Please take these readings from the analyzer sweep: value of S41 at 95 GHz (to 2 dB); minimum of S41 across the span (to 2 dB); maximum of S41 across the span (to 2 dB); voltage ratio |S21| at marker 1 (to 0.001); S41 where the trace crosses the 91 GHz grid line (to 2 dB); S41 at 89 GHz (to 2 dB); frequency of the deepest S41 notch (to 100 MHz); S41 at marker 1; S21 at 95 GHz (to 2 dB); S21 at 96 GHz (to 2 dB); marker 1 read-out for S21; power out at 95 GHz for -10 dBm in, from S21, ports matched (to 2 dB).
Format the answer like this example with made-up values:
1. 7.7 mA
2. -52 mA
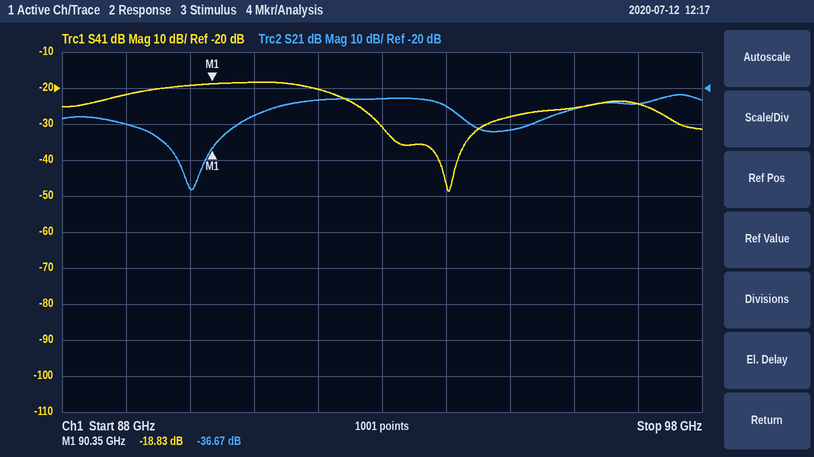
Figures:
1. -28 dB
2. -48 dB
3. -18 dB
4. 0.015
5. -18 dB
6. -22 dB
7. 94.0 GHz
8. -18.83 dB
9. -32 dB
10. -26 dB
11. -36.67 dB
12. -42 dBm
